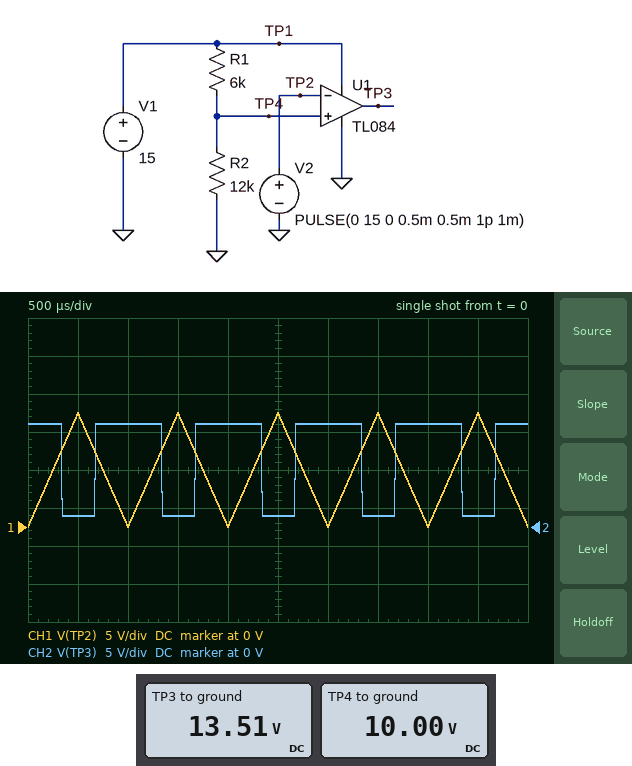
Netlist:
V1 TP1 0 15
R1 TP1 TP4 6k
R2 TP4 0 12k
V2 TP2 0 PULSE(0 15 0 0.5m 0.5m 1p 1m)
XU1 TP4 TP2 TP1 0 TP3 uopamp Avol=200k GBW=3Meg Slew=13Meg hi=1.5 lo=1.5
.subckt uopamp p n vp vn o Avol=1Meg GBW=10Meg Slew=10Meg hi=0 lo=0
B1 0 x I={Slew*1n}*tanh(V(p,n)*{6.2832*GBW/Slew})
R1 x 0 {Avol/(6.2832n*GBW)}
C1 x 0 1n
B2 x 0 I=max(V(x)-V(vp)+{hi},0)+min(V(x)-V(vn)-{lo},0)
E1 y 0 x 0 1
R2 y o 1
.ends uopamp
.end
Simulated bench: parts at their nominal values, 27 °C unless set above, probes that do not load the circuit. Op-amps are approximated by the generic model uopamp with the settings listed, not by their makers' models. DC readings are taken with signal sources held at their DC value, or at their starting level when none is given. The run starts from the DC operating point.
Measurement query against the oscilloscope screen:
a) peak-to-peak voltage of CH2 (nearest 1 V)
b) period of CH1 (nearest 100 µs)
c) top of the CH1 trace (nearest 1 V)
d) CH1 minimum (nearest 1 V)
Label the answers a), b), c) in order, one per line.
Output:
a) 12 V
b) 1.0 ms
c) 15 V
d) 0 V
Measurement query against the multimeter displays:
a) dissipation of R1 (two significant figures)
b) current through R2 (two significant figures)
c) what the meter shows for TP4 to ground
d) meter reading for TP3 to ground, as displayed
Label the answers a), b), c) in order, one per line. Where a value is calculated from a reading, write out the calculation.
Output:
a) (15 V - 10 V)^2 / 6 kΩ = 4.2 mW
b) (10 V) / 12 kΩ = 830 µA
c) 10.00 V
d) 13.51 V
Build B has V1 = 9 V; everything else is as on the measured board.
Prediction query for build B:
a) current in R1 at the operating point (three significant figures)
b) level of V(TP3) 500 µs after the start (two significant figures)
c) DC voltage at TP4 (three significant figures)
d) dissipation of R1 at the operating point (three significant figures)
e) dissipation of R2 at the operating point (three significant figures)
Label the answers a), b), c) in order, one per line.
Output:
a) 500 µA
b) 1.5 V
c) 6.00 V
d) 1.50 mW
e) 3.00 mW
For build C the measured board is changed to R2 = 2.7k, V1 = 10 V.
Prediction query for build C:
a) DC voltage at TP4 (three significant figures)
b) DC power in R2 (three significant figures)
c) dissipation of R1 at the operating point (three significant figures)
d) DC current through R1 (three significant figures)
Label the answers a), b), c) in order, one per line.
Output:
a) 3.10 V
b) 3.57 mW
c) 7.93 mW
d) 1.15 mA
